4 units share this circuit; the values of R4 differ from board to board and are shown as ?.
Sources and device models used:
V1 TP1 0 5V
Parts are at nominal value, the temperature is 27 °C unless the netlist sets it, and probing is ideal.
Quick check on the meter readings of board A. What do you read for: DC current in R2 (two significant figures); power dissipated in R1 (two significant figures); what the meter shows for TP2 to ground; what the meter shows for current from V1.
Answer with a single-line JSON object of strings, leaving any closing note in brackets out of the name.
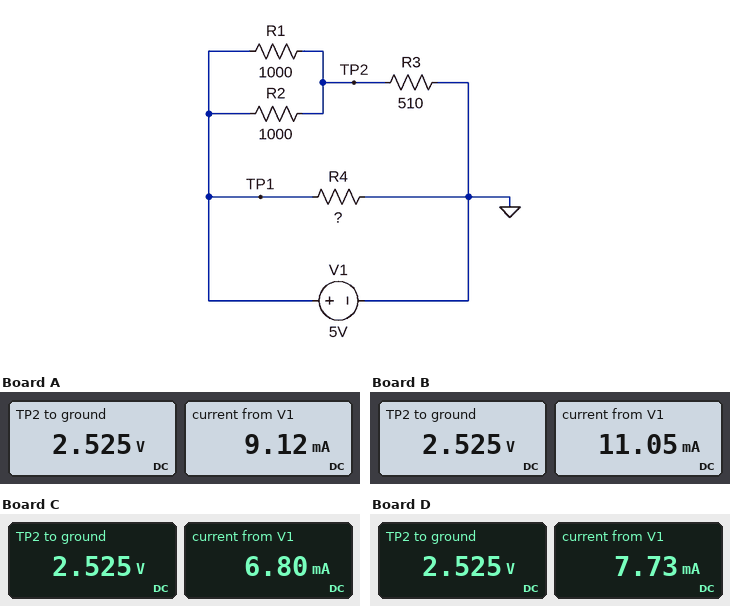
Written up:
{"DC current in R2": "2.5 mA", "power dissipated in R1": "6.1 mW", "what the meter shows for TP2 to ground": "2.525 V", "what the meter shows for current from V1": "9.12 mA"}
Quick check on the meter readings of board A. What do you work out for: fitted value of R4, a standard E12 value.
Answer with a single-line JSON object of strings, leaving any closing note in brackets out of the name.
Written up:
{"fitted value of R4, a standard E12 value": "1.2 kΩ"}
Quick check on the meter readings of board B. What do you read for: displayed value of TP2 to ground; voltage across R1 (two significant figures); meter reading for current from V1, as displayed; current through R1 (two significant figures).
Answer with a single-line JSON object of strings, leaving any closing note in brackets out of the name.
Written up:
{"displayed value of TP2 to ground": "2.525 V", "voltage across R1": "2.5 V", "meter reading for current from V1, as displayed": "11.05 mA", "current through R1": "2.5 mA"}
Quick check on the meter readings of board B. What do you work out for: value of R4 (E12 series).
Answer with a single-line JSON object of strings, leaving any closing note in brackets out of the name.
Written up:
{"value of R4": "820 Ω"}
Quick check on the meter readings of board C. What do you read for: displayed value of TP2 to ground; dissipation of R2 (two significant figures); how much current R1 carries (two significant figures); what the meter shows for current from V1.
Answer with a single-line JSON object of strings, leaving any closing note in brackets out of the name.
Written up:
{"displayed value of TP2 to ground": "2.525 V", "dissipation of R2": "6.1 mW", "how much current R1 carries": "2.5 mA", "what the meter shows for current from V1": "6.80 mA"}
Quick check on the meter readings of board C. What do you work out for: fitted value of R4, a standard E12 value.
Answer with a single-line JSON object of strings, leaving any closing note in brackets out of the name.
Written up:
{"fitted value of R4, a standard E12 value": "2.7 kΩ"}
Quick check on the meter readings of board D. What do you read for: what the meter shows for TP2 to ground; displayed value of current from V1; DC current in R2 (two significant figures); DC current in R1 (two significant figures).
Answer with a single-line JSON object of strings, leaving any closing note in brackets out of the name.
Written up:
{"what the meter shows for TP2 to ground": "2.525 V", "displayed value of current from V1": "7.73 mA", "DC current in R2": "2.5 mA", "DC current in R1": "2.5 mA"}
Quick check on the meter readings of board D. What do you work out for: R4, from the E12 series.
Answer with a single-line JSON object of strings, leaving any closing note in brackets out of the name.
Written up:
{"R4, from the E12 series": "1.8 kΩ"}
